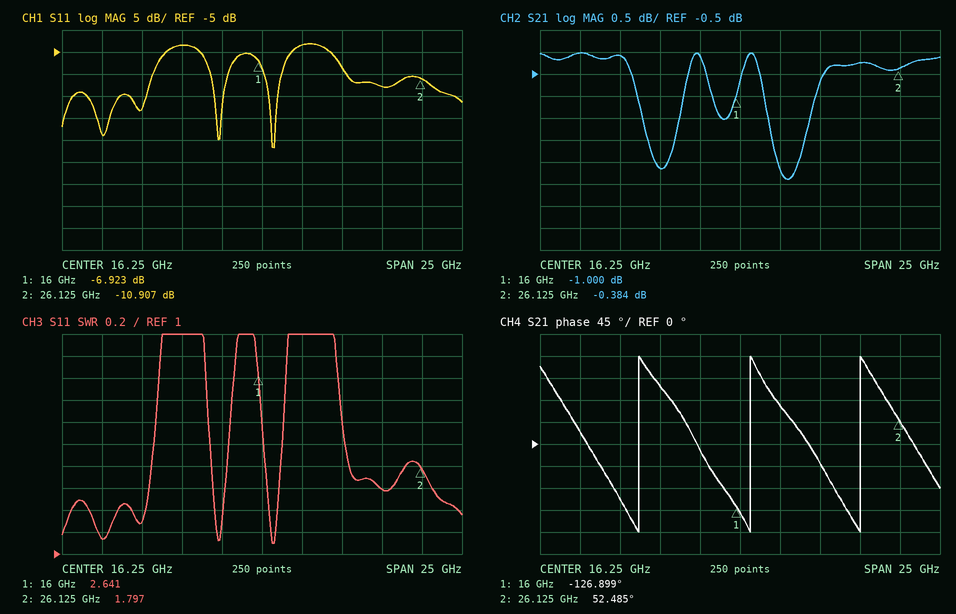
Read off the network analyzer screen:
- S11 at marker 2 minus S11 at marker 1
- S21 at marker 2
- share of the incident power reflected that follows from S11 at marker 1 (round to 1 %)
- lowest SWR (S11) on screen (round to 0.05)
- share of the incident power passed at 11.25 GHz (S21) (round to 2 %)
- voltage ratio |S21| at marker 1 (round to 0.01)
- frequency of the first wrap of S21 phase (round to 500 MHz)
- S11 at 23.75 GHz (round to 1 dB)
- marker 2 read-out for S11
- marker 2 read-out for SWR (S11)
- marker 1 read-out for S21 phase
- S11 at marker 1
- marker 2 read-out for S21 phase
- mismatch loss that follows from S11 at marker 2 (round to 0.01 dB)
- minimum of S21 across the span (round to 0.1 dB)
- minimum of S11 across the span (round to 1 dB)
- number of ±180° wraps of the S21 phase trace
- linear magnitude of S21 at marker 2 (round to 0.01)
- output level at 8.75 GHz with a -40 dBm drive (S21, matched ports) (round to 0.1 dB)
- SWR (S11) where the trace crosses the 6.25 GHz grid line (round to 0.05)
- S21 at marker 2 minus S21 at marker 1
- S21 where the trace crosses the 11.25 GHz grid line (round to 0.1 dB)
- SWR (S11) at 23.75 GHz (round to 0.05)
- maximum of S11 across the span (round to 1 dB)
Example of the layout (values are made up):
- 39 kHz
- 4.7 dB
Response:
- -3.984 dB
- -0.384 dB
- 20 %
- 1.10
- 54 %
- 0.89
- 10.0 GHz
- -13 dB
- -10.907 dB
- 1.797
- -126.899°
- -6.923 dB
- 52.485°
- 0.37 dB
- -2.9 dB
- -27 dB
- 3
- 0.96
- -40.1 dBm
- 1.15
- 0.616 dB
- -2.6 dB
- 1.60
- -3 dB
